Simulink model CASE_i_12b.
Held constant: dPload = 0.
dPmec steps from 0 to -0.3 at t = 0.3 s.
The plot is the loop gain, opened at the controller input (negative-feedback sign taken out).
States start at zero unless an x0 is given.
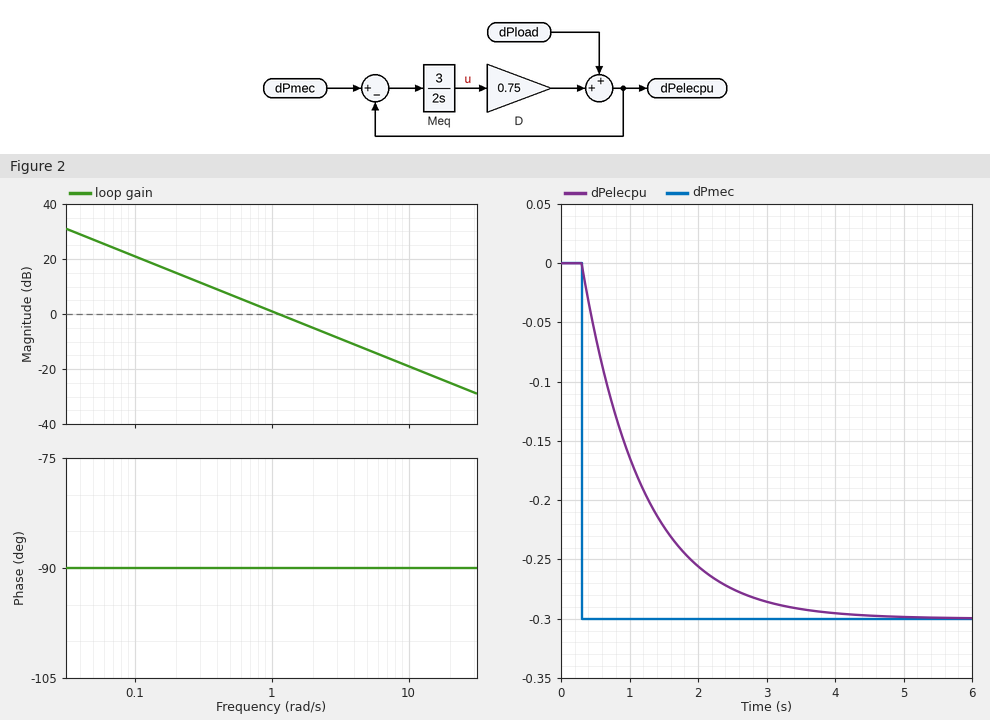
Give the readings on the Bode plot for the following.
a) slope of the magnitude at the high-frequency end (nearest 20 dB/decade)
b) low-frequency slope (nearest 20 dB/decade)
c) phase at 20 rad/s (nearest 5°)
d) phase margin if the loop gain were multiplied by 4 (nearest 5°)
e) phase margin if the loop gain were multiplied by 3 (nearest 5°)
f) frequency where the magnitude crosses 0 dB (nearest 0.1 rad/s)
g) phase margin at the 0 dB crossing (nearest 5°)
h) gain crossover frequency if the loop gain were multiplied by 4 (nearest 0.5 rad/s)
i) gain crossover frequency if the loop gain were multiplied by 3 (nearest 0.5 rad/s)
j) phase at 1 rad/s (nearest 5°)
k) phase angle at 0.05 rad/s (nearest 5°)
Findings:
-20 dB/decade
-20 dB/decade
-90°
90°
90°
1.1 rad/s
90°
4.5 rad/s
3.5 rad/s
-90°
-90°
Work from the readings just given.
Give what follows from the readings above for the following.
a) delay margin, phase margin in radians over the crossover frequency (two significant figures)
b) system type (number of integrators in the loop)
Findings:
1.4 s
1
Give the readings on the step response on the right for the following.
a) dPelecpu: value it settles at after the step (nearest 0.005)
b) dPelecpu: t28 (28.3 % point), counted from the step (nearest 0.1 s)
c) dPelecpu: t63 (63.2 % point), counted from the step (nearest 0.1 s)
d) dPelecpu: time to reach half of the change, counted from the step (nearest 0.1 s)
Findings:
-0.300
0.3 s
0.9 s
0.6 s
